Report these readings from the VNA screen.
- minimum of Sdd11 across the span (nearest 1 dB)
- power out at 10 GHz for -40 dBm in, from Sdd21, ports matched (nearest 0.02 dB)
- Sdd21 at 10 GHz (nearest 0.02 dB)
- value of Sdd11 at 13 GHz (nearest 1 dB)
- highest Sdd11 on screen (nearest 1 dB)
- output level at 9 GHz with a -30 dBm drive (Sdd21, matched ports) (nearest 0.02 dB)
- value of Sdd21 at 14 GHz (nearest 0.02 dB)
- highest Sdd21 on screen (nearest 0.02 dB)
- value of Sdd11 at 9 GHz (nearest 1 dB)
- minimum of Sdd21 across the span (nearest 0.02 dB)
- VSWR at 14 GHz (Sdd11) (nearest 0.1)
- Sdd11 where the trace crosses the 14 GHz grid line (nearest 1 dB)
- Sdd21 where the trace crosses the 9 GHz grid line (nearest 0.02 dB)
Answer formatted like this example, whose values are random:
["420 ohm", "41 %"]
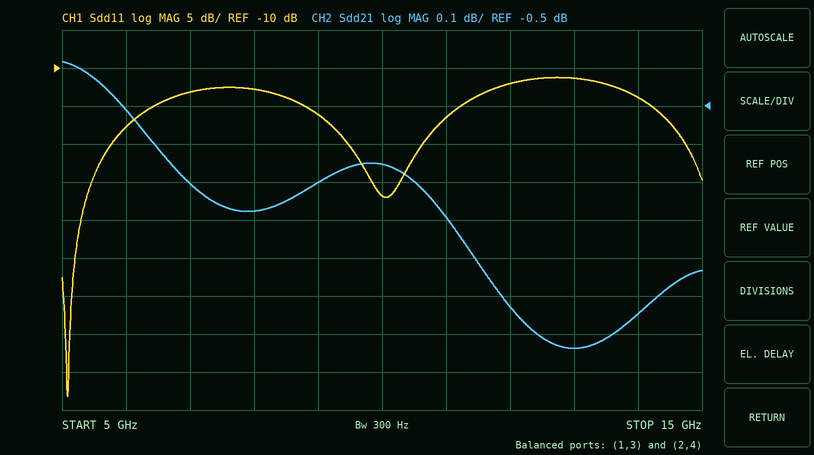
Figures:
["-53 dB", "-40.66 dBm", "-0.66 dB", "-11 dB", "-11 dB", "-30.70 dBm", "-1.04 dB", "-0.38 dB", "-16 dB", "-1.14 dB", "1.5", "-14 dB", "-0.70 dB"]
